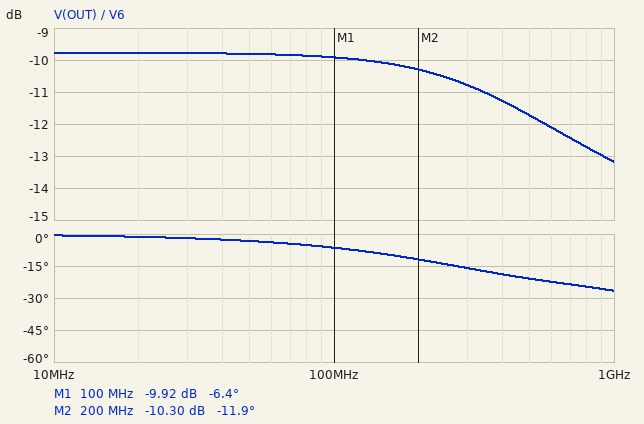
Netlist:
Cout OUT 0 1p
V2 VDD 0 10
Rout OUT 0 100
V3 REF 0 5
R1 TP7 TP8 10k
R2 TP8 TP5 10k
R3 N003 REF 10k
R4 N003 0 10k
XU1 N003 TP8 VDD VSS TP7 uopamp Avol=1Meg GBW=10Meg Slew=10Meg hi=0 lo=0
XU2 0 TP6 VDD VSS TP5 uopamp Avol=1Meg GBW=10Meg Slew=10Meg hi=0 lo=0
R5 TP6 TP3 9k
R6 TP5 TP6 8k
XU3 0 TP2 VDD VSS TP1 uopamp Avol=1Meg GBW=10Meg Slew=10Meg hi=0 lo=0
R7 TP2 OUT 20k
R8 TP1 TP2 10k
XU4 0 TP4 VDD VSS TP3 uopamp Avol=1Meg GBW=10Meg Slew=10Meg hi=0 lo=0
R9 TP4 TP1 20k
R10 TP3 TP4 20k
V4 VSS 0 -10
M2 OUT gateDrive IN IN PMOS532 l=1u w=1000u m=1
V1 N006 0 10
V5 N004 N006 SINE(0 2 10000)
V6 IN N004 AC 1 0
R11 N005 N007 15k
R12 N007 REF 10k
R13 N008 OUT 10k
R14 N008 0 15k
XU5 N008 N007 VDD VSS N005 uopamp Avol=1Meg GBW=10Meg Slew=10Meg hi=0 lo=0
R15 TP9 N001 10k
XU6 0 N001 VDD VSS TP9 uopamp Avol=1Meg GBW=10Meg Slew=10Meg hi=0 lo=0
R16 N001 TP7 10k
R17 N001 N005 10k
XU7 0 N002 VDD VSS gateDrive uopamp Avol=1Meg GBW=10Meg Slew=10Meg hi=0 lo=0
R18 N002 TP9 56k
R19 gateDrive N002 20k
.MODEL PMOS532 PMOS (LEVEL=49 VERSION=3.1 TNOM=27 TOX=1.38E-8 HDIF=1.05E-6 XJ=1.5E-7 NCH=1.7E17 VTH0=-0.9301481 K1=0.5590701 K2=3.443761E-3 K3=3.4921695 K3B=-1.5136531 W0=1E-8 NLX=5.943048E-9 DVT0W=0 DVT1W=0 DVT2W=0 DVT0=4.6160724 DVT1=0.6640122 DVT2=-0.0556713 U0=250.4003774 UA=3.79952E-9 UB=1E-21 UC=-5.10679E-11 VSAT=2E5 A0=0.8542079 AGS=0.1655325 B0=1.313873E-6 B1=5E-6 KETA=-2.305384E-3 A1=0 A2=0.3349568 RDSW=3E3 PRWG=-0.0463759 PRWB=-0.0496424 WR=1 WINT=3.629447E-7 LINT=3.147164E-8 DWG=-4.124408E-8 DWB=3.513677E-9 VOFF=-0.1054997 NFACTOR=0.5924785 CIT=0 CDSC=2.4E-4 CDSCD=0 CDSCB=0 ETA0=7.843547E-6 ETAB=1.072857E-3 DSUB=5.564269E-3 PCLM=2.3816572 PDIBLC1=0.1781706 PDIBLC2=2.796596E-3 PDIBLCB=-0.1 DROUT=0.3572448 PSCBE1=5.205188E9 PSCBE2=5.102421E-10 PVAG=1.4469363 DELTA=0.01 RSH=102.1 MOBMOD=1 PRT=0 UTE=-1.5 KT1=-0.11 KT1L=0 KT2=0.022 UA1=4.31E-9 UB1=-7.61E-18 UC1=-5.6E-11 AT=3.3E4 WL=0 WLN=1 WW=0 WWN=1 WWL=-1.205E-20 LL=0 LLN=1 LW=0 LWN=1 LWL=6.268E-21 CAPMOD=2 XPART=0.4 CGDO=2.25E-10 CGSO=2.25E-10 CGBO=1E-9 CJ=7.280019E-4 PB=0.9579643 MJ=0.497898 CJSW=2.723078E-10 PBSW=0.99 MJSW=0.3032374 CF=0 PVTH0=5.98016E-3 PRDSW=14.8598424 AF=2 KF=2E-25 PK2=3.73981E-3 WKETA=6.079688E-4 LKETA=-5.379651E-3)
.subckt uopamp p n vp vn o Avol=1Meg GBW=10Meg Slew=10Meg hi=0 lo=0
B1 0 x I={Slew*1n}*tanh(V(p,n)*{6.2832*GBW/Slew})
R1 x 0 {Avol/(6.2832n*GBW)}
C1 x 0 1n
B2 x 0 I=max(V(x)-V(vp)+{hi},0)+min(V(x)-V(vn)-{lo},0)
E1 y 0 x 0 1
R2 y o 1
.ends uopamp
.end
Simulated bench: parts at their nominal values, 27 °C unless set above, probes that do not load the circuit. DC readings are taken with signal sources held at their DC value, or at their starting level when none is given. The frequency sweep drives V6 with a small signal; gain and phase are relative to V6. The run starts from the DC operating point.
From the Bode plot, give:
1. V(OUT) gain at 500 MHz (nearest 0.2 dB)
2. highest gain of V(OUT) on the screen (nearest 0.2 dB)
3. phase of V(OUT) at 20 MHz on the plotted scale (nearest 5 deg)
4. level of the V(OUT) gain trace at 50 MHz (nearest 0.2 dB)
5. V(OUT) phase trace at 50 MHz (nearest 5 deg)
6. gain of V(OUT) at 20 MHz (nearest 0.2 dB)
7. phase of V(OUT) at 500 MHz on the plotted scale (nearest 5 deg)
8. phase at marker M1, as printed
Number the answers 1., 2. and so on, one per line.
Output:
1. -11.8 dB
2. -9.8 dB
3. 0 deg
4. -9.8 dB
5. -5 deg
6. -9.8 dB
7. -20 deg
8. -6.4 deg
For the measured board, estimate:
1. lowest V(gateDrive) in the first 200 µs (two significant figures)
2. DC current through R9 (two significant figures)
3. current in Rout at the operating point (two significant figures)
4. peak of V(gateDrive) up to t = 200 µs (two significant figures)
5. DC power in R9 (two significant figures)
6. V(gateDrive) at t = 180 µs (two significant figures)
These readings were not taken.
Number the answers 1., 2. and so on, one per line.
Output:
1. 830 mV
2. 78 µA
3. 31 mA
4. 1.7 V
5. 120 µW
6. 850 mV
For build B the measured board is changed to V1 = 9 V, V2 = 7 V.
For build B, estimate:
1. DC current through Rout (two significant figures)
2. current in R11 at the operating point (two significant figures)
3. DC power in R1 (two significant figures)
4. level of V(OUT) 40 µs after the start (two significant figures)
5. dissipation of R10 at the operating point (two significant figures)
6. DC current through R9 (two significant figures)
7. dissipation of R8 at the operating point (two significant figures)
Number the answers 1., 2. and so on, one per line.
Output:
1. 28 mA
2. 330 µA
3. 1.4 mW
4. 3.2 V
5. 98 µW
6. 70 µA
7. 200 µW
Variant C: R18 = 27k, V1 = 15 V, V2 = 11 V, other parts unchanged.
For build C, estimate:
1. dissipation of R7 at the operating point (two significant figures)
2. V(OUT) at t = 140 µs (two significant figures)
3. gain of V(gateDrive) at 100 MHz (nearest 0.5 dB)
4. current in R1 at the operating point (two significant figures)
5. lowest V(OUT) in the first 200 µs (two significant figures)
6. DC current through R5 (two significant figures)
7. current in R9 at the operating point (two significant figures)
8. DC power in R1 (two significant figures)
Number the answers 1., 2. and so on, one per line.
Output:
1. 1.1 mW
2. 5.0 V
3. -58.5 dB
4. 460 µA
5. 4.0 V
6. 260 µA
7. 120 µA
8. 2.1 mW
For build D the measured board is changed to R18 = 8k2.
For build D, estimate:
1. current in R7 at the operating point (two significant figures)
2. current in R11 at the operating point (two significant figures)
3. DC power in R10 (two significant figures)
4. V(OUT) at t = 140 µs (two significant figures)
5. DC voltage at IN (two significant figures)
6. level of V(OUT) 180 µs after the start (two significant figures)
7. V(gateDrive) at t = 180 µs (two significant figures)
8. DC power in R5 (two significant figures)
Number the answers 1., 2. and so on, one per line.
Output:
1. 120 µA
2. 360 µA
3. 68 µW
4. 2.5 V
5. 10 V
6. 2.0 V
7. 3.5 V
8. 150 µW
